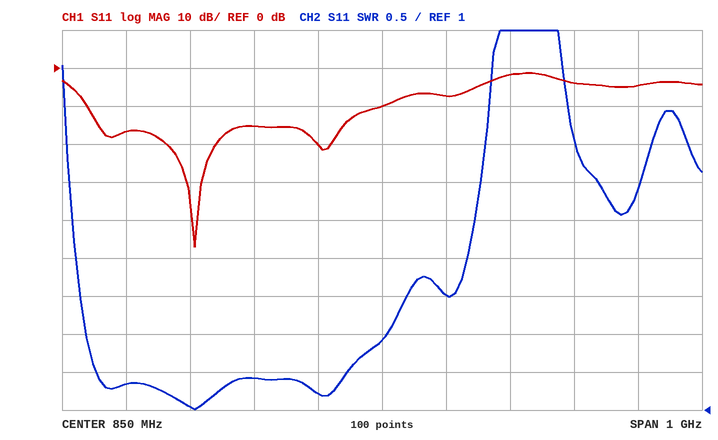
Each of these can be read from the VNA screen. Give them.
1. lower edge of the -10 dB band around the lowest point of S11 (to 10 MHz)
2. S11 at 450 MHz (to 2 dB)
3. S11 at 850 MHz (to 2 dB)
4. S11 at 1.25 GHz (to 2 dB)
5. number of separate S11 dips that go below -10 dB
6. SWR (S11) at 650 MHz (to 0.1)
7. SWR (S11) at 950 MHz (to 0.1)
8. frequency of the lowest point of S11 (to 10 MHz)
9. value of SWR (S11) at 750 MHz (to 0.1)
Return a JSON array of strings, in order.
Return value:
["390 MHz", "-16 dB", "-10 dB", "-4 dB", "2", "1.4", "2.5", "560 MHz", "1.2"]
